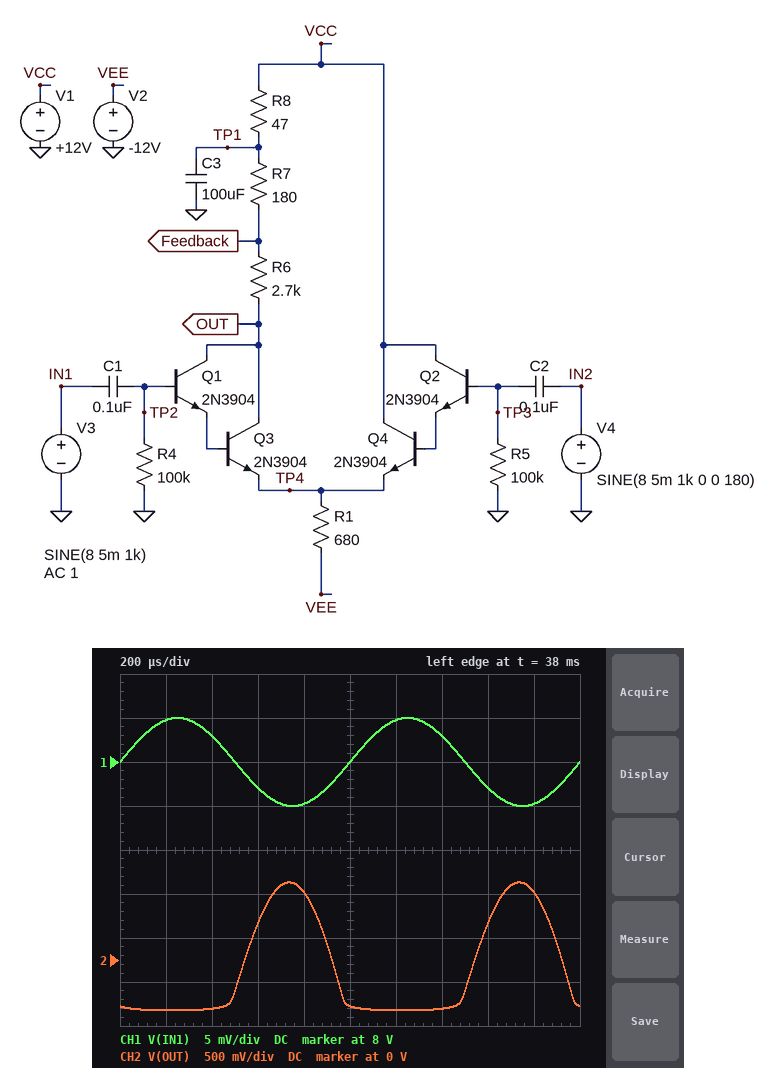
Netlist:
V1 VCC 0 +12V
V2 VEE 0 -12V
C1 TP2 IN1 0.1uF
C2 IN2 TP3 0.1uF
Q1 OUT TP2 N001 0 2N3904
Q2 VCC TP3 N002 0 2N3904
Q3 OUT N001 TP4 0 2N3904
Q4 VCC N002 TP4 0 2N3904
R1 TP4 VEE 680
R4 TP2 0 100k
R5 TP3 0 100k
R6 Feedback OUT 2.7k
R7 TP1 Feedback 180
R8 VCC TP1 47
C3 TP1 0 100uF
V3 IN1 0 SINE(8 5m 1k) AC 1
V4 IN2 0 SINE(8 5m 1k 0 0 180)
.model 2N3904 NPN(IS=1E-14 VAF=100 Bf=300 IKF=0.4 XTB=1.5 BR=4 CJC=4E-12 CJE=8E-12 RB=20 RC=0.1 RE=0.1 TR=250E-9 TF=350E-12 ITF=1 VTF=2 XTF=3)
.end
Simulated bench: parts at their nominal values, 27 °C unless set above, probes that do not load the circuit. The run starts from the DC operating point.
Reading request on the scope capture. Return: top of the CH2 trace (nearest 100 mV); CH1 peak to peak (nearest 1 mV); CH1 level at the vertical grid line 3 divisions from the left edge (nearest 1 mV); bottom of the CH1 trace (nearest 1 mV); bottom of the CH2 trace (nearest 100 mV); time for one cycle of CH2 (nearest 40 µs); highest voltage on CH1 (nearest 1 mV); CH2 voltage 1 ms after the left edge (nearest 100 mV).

900 mV
10 mV
7.997 V
7.995 V
-600 mV
1.00 ms
8.005 V
-500 mV
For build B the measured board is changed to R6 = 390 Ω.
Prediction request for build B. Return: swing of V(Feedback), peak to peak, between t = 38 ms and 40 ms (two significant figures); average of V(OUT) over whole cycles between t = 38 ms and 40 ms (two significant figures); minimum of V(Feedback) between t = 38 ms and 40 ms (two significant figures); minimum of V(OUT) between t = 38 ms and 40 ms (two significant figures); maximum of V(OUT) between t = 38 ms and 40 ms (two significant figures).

250 mV
7.3 V
10 V
6.9 V
7.7 V
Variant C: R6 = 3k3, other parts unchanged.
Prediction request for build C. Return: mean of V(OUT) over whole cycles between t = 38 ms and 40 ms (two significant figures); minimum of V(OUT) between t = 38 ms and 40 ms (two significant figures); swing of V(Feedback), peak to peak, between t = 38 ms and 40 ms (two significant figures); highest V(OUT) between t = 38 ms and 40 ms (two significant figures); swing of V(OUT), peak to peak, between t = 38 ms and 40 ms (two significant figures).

-250 mV
-590 mV
60 mV
580 mV
1.2 V
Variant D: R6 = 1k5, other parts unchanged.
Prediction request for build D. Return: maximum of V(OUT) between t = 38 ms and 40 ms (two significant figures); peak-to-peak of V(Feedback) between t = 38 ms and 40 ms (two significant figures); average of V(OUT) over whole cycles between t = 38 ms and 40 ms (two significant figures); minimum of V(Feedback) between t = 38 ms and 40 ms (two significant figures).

1.4 V
210 mV
390 mV
10 V
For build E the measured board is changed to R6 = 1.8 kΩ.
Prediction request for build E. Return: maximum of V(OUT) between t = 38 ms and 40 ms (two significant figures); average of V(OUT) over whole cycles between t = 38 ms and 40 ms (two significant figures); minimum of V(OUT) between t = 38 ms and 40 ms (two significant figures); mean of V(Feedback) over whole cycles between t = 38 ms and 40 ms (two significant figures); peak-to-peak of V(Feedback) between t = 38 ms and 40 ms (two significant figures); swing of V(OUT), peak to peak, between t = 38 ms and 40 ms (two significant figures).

1.3 V
230 mV
-540 mV
11 V
170 mV
1.8 V
